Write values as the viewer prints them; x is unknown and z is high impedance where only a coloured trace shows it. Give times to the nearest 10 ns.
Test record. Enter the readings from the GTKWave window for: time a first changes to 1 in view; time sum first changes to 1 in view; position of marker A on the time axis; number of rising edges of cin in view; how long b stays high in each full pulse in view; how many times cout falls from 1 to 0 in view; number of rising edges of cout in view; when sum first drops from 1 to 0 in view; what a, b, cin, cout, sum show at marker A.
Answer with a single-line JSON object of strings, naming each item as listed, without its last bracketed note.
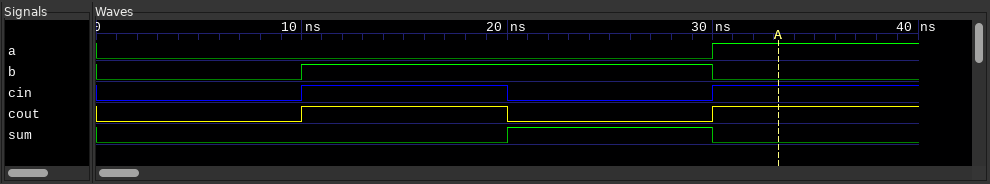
{"time a first changes to 1 in view": "30 ns", "time sum first changes to 1 in view": "20 ns", "position of marker A on the time axis": "30 ns", "number of rising edges of cin in view": "2", "how long b stays high in each full pulse in view": "20 ns", "how many times cout falls from 1 to 0 in view": "1", "number of rising edges of cout in view": "2", "when sum first drops from 1 to 0 in view": "30 ns", "what a, b, cin, cout, sum show at marker A": "a=1, b=0, cin=1, cout=1, sum=0"}
